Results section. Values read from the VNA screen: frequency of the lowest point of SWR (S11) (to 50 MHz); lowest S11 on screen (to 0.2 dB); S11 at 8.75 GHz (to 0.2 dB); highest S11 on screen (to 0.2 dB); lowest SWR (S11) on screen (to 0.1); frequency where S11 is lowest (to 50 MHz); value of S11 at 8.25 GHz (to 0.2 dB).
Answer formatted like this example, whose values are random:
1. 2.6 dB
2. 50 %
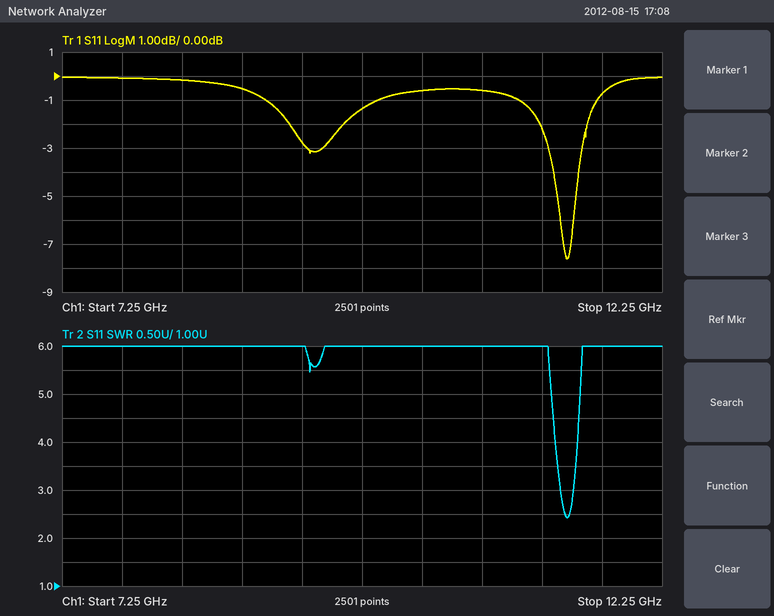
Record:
1. 11.45 GHz
2. -7.6 dB
3. -0.6 dB
4. 0.0 dB
5. 2.4
6. 11.45 GHz
7. -0.2 dB
